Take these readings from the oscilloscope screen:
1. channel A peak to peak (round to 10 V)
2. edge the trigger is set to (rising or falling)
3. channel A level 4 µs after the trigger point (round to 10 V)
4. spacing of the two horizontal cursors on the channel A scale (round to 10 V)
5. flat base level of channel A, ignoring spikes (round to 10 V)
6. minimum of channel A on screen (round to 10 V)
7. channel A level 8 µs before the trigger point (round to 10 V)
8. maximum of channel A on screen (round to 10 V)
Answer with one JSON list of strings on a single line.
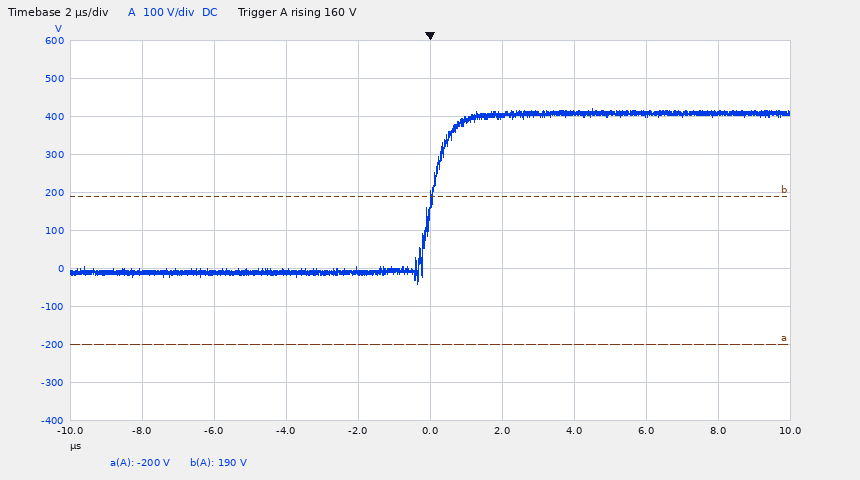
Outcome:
["460 V", "rising", "410 V", "390 V", "-10 V", "-40 V", "-10 V", "420 V"]
